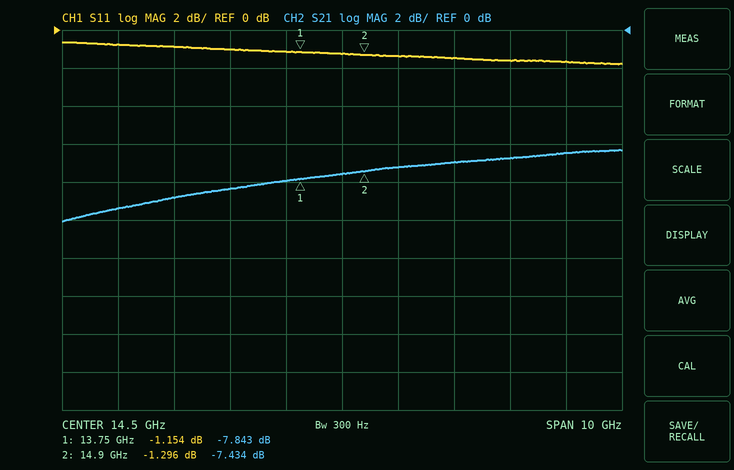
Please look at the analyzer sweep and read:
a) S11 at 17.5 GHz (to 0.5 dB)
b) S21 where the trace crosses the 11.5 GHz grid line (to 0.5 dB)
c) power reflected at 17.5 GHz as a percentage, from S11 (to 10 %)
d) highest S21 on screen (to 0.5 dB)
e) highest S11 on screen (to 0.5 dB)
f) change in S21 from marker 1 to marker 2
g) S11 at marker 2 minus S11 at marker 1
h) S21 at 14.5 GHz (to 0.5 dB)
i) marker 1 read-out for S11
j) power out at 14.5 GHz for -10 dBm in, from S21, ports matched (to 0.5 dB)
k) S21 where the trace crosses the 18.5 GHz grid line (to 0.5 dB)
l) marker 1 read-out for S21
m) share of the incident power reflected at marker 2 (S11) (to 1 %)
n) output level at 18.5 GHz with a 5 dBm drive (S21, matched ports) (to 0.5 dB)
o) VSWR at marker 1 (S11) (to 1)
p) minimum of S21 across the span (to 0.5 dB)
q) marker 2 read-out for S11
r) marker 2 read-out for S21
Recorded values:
-1.5 dB
-9.0 dB
70 %
-6.5 dB
-0.5 dB
0.409 dB
-0.142 dB
-7.5 dB
-1.154 dB
-17.5 dBm
-6.5 dB
-7.843 dB
74 %
-1.5 dBm
15
-10.0 dB
-1.296 dB
-7.434 dB
